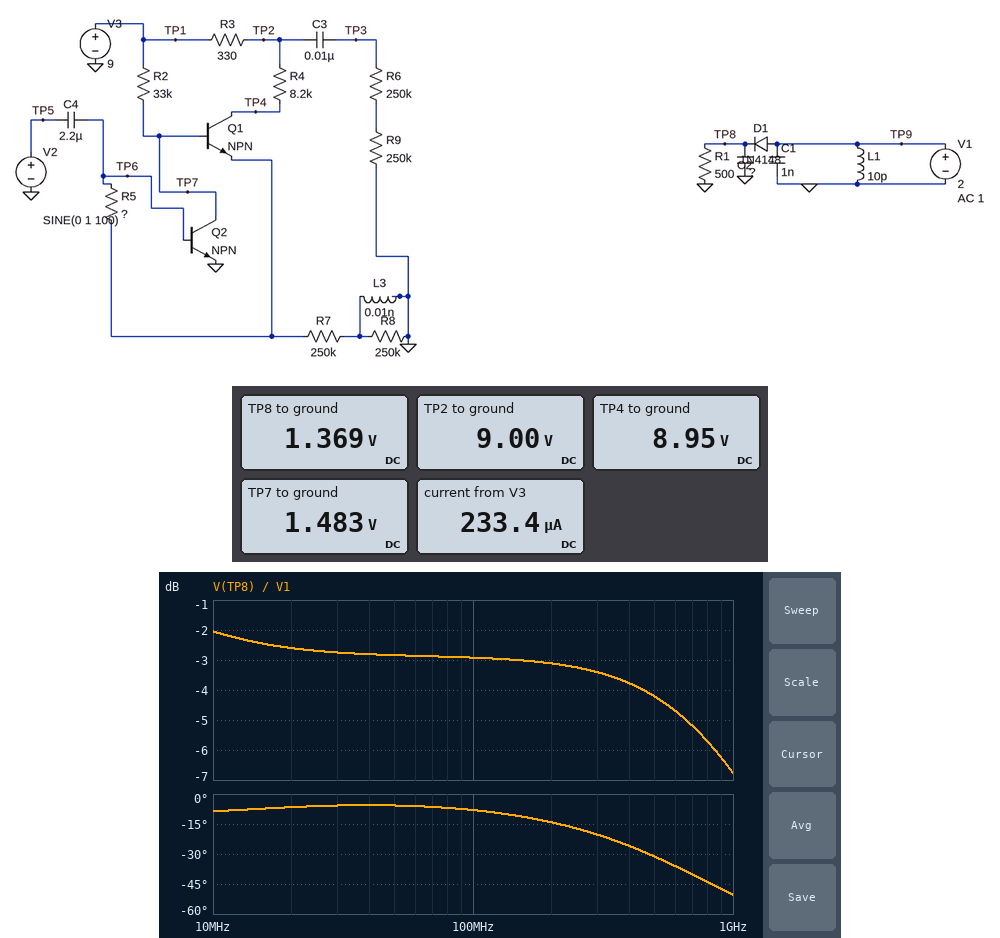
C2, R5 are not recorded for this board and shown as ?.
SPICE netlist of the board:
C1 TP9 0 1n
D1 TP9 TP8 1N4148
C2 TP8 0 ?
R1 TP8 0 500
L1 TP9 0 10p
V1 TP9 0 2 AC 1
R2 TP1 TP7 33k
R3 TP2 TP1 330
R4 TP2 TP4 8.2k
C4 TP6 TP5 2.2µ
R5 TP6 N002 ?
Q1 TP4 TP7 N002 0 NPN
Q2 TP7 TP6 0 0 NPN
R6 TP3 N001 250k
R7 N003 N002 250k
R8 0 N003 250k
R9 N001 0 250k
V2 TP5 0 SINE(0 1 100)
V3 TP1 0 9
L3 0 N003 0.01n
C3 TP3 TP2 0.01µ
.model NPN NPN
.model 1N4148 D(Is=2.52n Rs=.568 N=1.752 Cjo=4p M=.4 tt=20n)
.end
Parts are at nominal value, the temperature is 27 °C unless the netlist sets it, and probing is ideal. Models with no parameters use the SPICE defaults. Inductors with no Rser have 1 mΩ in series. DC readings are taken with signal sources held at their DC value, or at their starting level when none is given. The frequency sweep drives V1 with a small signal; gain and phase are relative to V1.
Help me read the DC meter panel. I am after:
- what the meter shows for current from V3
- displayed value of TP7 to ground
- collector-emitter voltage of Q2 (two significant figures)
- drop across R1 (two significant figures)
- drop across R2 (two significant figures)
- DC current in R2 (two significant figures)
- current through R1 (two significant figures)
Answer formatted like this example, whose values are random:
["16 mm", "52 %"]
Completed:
["233.4 µA", "1.483 V", "1.5 V", "1.4 V", "7.5 V", "230 µA", "2.7 mA"]
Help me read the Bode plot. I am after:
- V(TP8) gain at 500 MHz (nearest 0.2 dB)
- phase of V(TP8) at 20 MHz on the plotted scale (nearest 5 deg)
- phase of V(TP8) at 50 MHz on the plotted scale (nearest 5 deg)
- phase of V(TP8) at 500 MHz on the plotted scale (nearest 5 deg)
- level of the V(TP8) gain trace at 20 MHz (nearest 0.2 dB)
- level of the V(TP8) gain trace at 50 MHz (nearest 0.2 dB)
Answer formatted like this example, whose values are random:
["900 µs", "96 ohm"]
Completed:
["-4.2 dB", "-5 deg", "-5 deg", "-30 deg", "-2.6 dB", "-2.8 dB"]
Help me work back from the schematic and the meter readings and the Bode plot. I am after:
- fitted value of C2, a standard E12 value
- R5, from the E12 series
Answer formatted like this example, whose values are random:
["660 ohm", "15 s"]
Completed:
["470 pF", "47 kΩ"]
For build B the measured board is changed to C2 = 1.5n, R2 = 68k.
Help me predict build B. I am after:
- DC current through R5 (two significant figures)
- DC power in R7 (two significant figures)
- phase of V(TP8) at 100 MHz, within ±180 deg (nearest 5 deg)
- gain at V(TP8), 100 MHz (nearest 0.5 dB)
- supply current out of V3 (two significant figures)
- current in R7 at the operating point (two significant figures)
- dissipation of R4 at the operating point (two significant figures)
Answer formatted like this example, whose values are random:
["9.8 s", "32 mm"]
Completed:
["1.1 µA", "2.4 µW", "-15 deg", "-7.5 dB", "120 µA", "3.1 µA", "140 nW"]
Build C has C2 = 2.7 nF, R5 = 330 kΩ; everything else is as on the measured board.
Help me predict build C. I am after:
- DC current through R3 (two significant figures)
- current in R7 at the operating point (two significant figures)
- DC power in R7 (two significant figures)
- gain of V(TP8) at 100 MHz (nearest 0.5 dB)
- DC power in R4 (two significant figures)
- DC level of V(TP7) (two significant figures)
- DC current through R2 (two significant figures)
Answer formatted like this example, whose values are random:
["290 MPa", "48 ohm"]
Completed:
["7.7 µA", "5.7 µA", "8.1 µW", "-10.5 dB", "490 nW", "2.1 V", "210 µA"]
